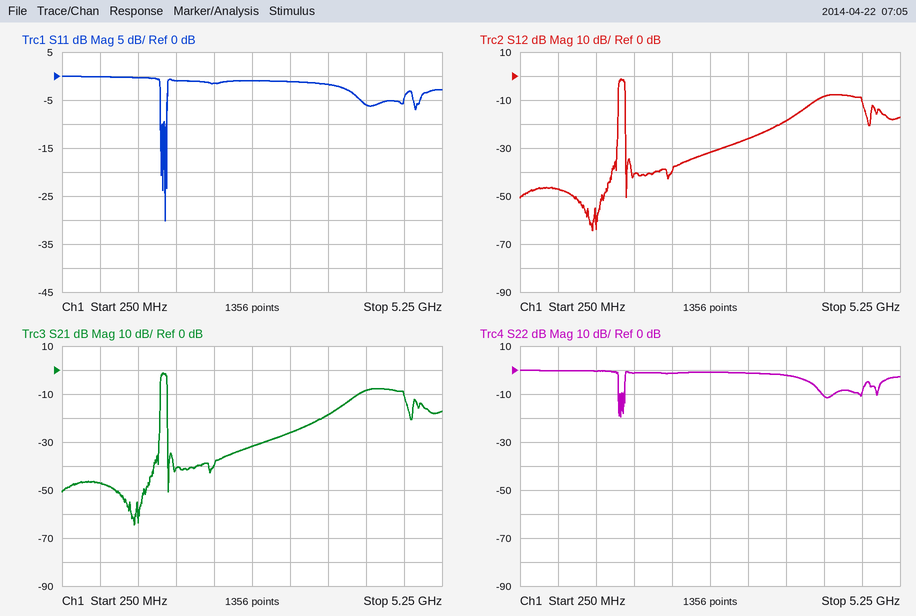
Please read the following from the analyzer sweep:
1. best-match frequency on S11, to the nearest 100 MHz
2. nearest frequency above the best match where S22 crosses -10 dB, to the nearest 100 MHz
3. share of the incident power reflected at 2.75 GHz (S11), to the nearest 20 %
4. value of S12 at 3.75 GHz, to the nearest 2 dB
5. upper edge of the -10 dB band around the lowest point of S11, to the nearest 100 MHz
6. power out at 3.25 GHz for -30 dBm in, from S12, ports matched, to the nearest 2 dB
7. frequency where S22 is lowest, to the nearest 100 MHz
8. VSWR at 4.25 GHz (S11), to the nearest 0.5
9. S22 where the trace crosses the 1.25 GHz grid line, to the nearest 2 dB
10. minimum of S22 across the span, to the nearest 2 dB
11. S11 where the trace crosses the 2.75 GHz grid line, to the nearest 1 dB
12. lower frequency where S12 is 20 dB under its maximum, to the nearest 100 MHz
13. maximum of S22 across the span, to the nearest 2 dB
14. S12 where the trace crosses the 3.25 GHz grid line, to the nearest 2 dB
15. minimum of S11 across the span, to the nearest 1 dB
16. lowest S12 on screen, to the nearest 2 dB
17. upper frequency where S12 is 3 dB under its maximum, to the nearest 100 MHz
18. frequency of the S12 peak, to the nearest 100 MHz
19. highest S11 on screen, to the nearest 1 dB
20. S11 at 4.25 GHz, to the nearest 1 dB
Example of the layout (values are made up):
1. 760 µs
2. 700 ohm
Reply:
1. 1.6 GHz
2. 1.6 GHz
3. 80 %
4. -18 dB
5. 1.6 GHz
6. -56 dBm
7. 1.6 GHz
8. 3.0
9. 0 dB
10. -20 dB
11. -1 dB
12. 1.5 GHz
13. 0 dB
14. -26 dB
15. -30 dB
16. -64 dB
17. 1.6 GHz
18. 1.6 GHz
19. 0 dB
20. -6 dB
